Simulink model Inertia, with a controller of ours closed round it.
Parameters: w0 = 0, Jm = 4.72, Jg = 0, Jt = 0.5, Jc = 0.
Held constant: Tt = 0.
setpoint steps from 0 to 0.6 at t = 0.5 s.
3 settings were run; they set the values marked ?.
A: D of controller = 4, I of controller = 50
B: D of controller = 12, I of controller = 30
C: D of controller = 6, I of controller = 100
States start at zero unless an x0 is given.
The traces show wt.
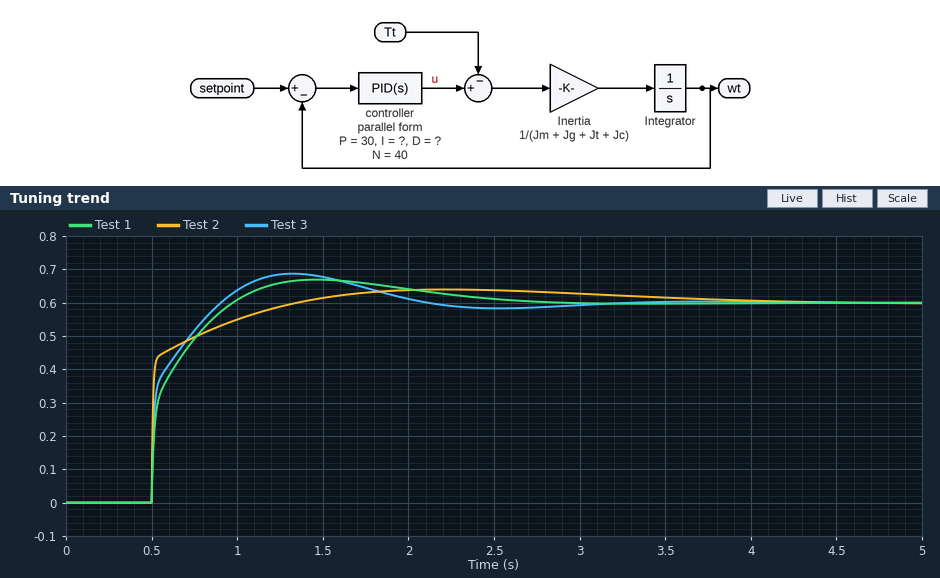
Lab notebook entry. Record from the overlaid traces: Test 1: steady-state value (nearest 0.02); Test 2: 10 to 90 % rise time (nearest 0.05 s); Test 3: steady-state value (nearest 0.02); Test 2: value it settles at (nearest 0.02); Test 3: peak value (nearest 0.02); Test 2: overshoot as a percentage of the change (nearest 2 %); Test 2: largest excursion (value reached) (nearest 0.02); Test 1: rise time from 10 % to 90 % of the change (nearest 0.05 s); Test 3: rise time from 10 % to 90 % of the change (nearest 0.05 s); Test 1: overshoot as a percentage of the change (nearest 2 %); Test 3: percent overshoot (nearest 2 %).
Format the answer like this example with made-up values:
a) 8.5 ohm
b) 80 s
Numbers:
a) 0.60
b) 0.45 s
c) 0.60
d) 0.60
e) 0.68
f) 6 %
g) 0.64
h) 0.35 s
i) 0.30 s
j) 12 %
k) 14 %
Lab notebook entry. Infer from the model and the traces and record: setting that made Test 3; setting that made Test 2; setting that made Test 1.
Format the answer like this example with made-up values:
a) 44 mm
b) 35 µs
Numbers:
a) C
b) B
c) A
